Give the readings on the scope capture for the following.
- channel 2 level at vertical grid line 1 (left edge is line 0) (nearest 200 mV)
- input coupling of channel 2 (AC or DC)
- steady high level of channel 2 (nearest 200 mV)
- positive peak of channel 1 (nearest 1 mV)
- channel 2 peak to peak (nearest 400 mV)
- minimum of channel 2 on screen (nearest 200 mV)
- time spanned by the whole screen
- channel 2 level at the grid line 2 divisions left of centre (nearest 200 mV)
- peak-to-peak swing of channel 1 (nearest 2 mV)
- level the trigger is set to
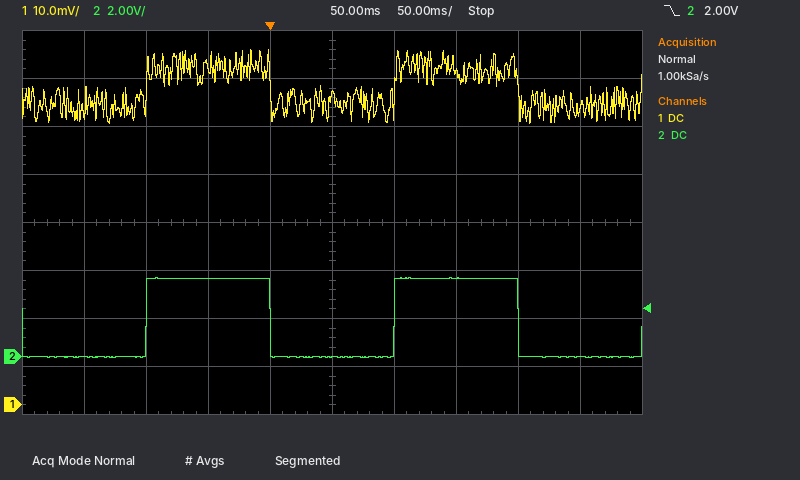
0.0 V
DC
3.2 V
74 mV
3.2 V
0.0 V
500 ms
3.2 V
16 mV
2.00 V
